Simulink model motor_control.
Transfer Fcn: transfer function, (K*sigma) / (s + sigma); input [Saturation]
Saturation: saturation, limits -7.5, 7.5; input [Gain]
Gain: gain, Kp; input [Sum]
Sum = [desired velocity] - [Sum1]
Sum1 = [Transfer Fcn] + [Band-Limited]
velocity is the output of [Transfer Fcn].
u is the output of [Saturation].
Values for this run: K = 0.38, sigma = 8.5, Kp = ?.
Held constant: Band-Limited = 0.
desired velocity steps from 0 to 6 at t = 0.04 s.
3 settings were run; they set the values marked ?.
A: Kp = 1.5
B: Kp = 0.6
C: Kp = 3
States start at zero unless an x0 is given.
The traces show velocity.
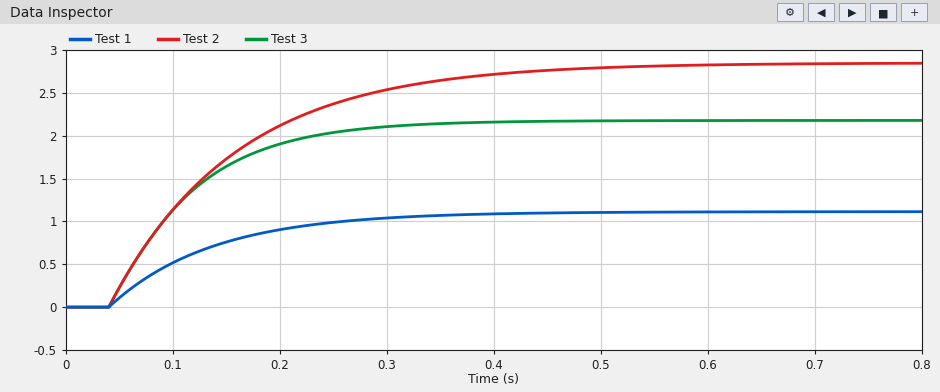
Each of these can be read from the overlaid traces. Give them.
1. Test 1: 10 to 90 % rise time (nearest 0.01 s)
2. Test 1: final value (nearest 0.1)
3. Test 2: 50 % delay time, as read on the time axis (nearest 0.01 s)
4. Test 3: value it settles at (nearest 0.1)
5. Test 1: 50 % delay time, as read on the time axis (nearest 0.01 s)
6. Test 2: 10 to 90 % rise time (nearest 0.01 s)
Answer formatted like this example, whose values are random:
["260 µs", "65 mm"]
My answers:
["0.21 s", "1.1", "0.12 s", "2.2", "0.11 s", "0.26 s"]
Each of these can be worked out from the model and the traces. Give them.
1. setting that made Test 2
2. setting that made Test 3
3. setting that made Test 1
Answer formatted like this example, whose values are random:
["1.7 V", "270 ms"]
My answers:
["C", "A", "B"]
